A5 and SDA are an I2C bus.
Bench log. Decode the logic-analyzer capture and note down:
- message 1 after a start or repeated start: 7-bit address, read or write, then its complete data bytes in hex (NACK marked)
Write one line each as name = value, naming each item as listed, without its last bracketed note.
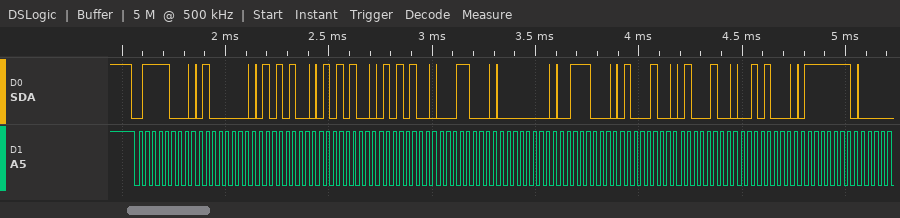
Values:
message 1 after a start or repeated start: 7-bit address, read or write, then its complete data bytes in hex = 0x3C write: 40 54 54 54 18 00 38 44 44 28 7F
